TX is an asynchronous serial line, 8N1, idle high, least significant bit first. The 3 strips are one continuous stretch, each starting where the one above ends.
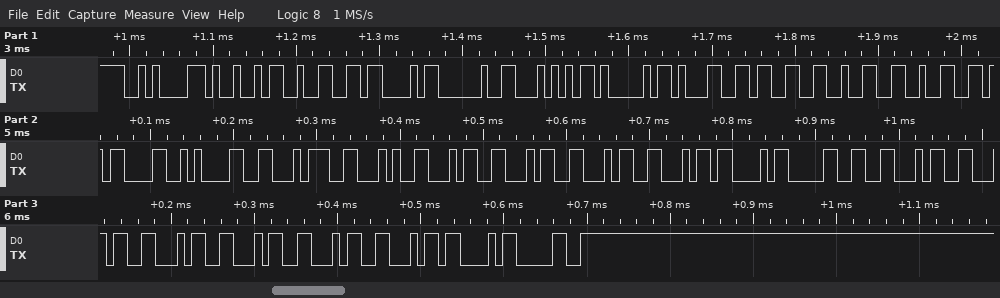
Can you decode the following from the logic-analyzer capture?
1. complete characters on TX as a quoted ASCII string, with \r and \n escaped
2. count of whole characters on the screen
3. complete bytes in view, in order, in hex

"\nI2C TA1322\r\nFFFFFFC0FFFFFFC0"
29
0A 49 32 43 20 54 41 31 33 32 32 0D 0A 46 46 46 46 46 46 43 30 46 46 46 46 46 46 43 30
